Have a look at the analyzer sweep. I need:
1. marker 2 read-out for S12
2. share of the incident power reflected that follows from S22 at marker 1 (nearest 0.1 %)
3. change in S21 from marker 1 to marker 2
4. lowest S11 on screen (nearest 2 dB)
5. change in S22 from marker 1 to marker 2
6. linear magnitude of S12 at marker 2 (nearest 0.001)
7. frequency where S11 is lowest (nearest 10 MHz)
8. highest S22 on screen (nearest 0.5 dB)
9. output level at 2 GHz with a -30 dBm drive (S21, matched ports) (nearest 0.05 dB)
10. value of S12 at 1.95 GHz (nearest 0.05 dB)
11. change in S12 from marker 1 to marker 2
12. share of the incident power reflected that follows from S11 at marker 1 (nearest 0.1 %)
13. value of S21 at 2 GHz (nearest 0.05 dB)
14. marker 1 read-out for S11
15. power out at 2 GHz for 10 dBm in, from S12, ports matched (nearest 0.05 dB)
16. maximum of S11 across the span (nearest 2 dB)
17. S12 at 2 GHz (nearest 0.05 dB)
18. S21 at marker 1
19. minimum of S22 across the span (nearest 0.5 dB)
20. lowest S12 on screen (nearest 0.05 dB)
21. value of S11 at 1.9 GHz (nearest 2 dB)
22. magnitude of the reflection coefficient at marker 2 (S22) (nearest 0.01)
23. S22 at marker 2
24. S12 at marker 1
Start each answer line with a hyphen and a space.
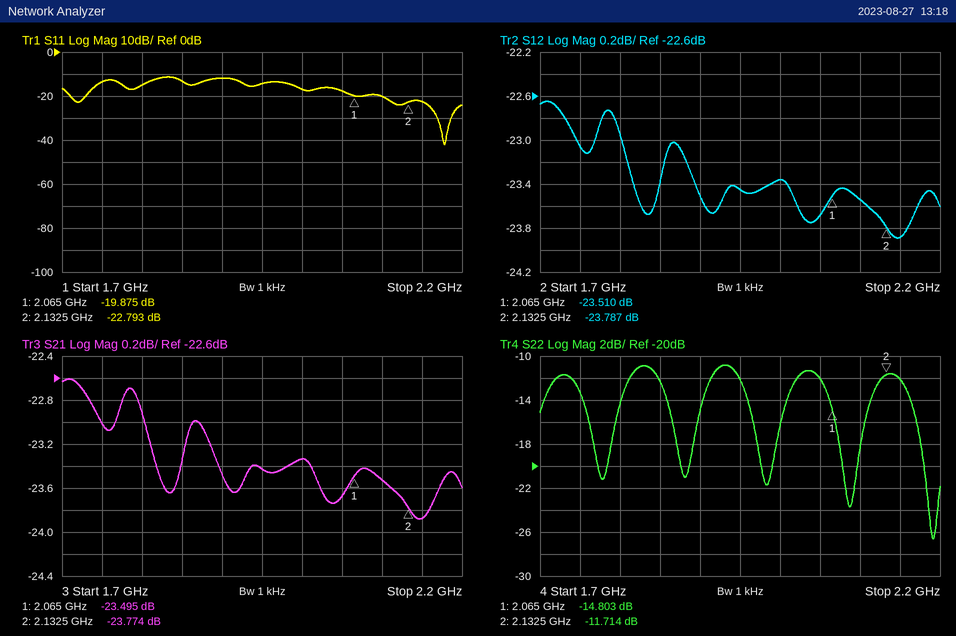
- -23.787 dB
- 3.3 %
- -0.279 dB
- -42 dB
- 3.089 dB
- 0.065
- 2.18 GHz
- -11.0 dB
- -53.35 dBm
- -23.45 dB
- -0.277 dB
- 1.0 %
- -23.35 dB
- -19.875 dB
- -13.35 dBm
- -12 dB
- -23.35 dB
- -23.495 dB
- -26.5 dB
- -23.90 dB
- -12 dB
- 0.26
- -11.714 dB
- -23.510 dB
